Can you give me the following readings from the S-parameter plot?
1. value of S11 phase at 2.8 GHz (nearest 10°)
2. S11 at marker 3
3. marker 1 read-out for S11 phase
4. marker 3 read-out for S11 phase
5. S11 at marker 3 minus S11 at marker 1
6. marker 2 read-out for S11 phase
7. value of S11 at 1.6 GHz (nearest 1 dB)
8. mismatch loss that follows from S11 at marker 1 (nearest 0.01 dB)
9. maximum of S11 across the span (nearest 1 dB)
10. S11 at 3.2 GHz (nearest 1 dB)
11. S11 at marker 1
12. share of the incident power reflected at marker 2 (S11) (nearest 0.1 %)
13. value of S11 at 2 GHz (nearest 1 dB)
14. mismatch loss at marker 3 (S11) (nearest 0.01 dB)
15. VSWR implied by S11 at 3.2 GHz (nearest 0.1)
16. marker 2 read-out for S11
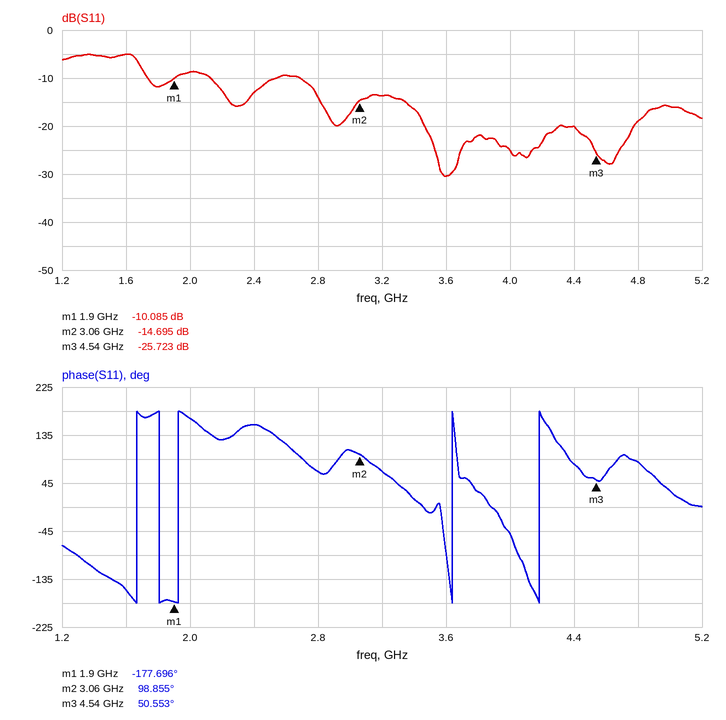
70°
-25.723 dB
-177.696°
50.553°
-15.638 dB
98.855°
-5 dB
0.45 dB
-5 dB
-14 dB
-10.085 dB
3.4 %
-9 dB
0.01 dB
1.5
-14.695 dB
